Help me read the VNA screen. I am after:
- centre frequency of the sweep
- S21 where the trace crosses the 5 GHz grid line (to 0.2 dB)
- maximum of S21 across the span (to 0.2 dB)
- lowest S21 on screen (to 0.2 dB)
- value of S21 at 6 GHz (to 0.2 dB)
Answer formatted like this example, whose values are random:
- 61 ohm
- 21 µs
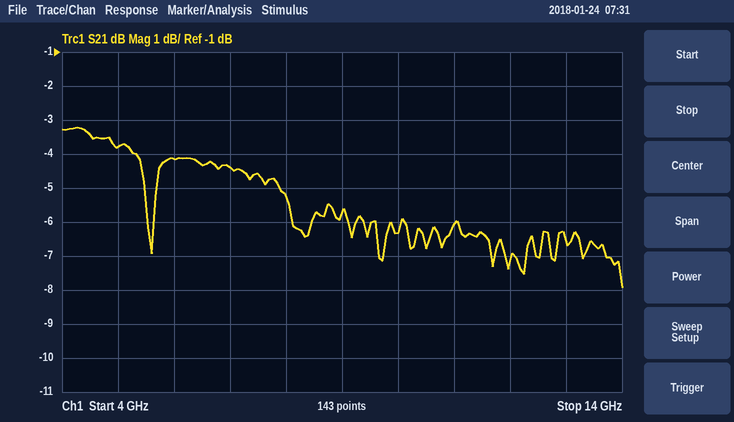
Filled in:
- 9 GHz
- -3.8 dB
- -3.2 dB
- -8.0 dB
- -4.2 dB
